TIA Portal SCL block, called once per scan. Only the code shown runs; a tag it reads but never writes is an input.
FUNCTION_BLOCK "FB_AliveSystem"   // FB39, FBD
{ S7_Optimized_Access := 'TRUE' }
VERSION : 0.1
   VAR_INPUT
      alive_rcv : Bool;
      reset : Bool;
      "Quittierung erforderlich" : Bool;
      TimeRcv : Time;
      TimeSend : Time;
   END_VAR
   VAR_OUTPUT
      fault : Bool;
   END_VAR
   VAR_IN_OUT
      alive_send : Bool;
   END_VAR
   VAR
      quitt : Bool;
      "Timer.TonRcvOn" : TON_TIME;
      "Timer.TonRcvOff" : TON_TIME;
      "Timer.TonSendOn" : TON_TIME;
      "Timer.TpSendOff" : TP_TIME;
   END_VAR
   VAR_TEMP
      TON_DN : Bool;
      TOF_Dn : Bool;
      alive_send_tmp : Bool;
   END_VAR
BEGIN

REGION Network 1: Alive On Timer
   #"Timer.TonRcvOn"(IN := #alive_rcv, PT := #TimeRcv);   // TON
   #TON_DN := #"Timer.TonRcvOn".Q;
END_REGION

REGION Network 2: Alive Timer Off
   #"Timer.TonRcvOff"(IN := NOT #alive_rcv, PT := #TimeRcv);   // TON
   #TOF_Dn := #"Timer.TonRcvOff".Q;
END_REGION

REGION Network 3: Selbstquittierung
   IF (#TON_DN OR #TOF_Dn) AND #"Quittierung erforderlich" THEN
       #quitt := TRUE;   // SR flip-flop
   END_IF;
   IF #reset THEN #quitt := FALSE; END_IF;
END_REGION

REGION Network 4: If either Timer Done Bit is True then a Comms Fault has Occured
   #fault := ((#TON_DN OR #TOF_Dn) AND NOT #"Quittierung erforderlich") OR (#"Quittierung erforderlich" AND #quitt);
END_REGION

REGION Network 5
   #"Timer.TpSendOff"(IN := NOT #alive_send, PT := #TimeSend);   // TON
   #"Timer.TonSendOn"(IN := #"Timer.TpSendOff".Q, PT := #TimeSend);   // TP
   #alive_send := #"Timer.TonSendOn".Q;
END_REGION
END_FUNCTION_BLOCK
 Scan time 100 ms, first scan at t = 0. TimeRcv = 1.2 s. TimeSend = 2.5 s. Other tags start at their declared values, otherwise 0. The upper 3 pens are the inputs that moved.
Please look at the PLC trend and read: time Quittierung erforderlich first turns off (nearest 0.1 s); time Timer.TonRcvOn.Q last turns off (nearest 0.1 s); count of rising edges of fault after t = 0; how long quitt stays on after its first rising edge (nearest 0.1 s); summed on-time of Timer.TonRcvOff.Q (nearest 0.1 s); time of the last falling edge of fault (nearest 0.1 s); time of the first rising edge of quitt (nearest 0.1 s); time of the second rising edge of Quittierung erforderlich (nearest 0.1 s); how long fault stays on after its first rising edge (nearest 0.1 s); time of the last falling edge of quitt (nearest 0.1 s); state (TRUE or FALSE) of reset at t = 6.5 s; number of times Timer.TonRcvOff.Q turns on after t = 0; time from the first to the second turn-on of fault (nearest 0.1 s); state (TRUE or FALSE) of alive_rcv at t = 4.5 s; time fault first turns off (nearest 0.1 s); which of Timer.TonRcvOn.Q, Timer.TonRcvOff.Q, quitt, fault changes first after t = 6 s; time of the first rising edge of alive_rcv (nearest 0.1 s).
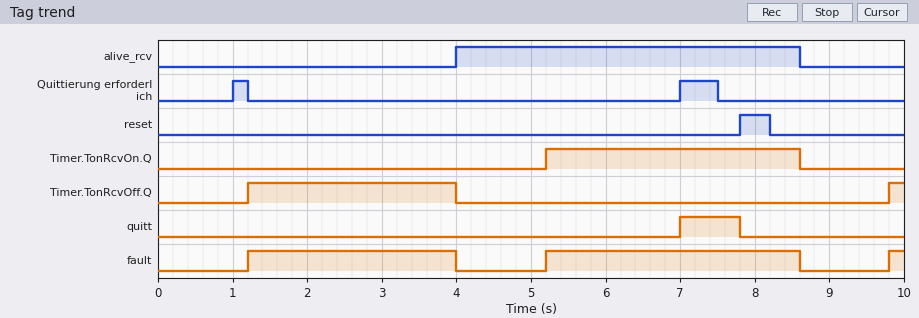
1.2 s
8.6 s
3
0.8 s
3.0 s
8.6 s
7.0 s
7.0 s
2.8 s
7.8 s
FALSE
2
4.0 s
TRUE
4.0 s
quitt
4.0 s
